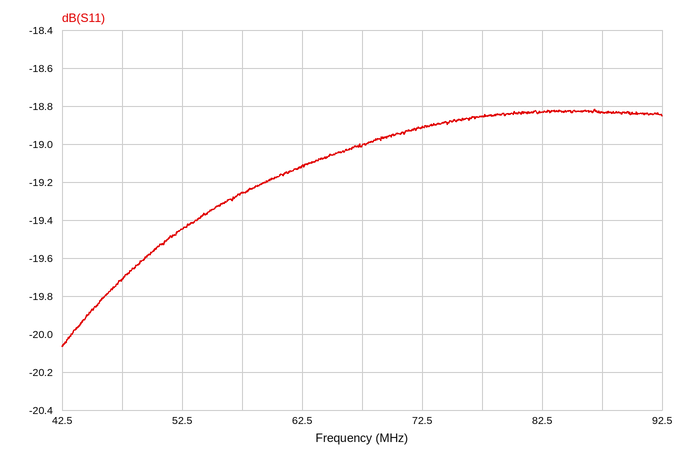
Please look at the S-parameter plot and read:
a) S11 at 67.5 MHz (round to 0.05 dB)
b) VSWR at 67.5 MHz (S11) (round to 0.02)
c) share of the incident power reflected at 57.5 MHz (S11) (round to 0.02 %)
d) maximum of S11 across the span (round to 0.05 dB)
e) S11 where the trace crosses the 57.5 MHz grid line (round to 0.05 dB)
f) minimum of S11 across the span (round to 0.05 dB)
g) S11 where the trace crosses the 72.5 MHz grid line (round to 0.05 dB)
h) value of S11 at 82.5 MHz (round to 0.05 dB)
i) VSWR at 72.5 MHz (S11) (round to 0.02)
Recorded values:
-19.00 dB
1.26
1.18 %
-18.80 dB
-19.25 dB
-20.05 dB
-18.90 dB
-18.85 dB
1.26
